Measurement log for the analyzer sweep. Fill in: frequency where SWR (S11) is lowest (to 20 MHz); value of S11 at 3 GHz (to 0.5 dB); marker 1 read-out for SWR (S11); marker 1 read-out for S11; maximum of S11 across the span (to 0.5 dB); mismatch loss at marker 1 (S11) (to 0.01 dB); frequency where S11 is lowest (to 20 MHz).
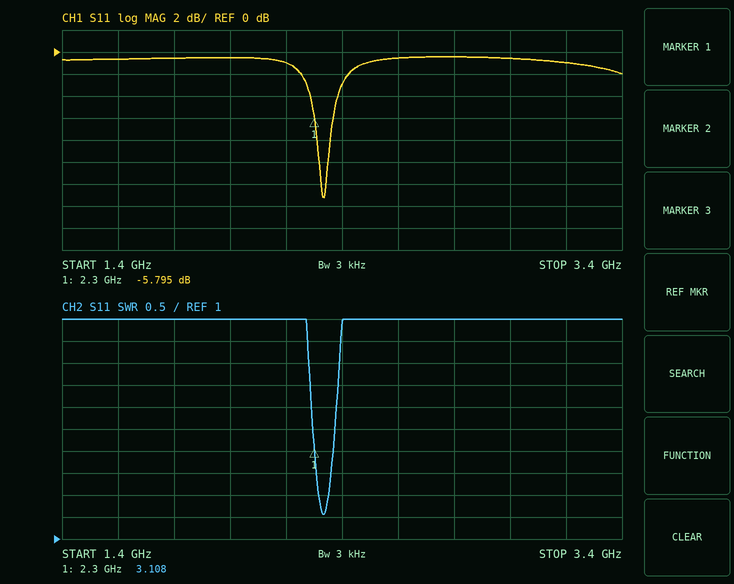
2.34 GHz
-0.5 dB
3.108
-5.795 dB
-0.5 dB
1.33 dB
2.34 GHz
